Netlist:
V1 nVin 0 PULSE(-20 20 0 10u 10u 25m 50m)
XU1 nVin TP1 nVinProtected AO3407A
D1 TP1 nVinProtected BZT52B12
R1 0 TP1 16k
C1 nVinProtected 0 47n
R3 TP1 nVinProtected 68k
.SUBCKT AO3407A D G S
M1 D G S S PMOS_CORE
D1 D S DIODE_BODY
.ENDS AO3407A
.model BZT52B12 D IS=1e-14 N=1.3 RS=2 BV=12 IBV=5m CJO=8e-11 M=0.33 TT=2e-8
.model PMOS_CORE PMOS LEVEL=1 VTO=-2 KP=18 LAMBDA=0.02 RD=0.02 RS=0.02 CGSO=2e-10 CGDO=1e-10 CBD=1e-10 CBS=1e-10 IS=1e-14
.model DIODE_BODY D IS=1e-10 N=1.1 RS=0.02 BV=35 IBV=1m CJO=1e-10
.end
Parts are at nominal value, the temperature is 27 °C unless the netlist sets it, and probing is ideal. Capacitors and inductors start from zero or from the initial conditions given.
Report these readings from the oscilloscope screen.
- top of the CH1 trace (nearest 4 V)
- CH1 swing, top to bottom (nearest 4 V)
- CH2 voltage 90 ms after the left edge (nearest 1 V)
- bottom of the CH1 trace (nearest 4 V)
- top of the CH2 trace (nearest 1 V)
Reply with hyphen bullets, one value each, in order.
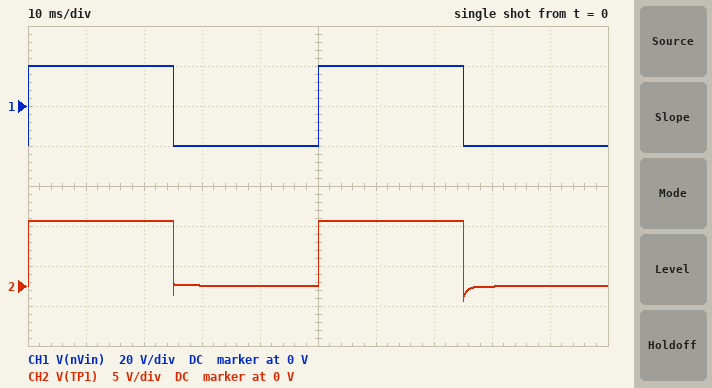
- 20 V
- 40 V
- 0 V
- -20 V
- 8 V
